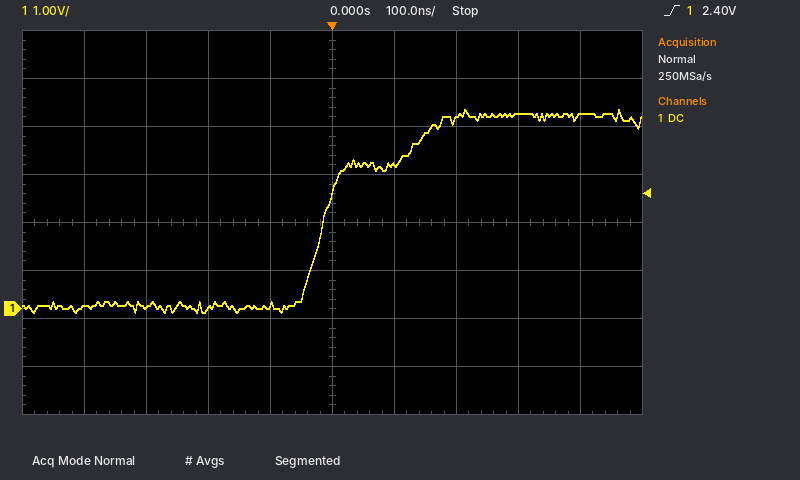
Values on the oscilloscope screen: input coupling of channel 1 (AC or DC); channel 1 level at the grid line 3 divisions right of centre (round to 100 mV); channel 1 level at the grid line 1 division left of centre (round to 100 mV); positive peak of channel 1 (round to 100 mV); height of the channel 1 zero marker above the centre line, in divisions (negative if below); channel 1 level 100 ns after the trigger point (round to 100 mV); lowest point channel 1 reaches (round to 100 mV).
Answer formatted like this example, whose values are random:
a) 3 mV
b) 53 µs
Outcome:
a) DC
b) 4.1 V
c) 100 mV
d) 4.2 V
e) -1.8 div
f) 3.0 V
g) -100 mV
